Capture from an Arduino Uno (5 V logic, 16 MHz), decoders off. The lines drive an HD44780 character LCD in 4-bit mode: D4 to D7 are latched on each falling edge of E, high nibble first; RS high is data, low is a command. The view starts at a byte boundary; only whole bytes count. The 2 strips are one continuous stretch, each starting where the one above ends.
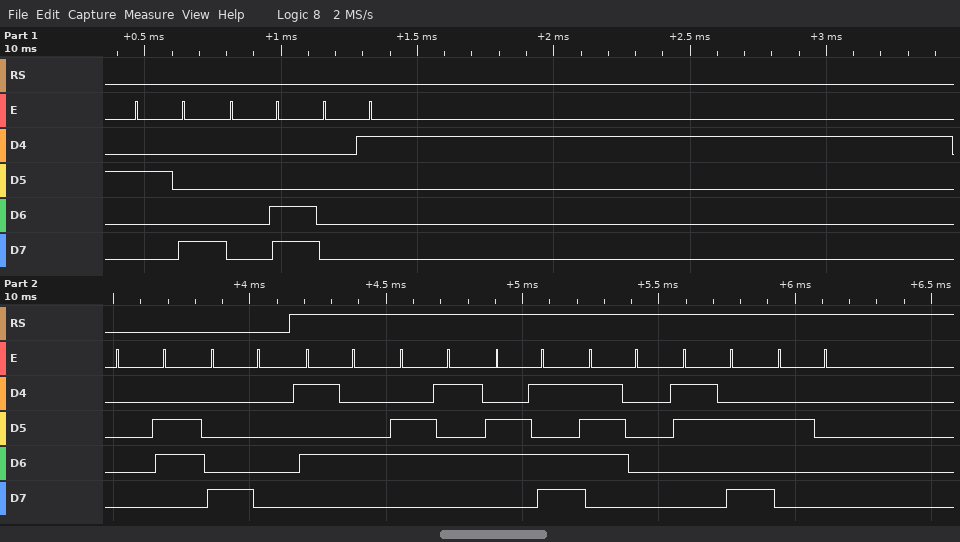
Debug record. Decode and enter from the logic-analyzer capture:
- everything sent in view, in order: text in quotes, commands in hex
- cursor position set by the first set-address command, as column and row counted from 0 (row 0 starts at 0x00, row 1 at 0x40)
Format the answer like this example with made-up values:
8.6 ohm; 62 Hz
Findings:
0x28 0x0C 0x01 0x06 0x80 "Temp: "; column 0, row 0
